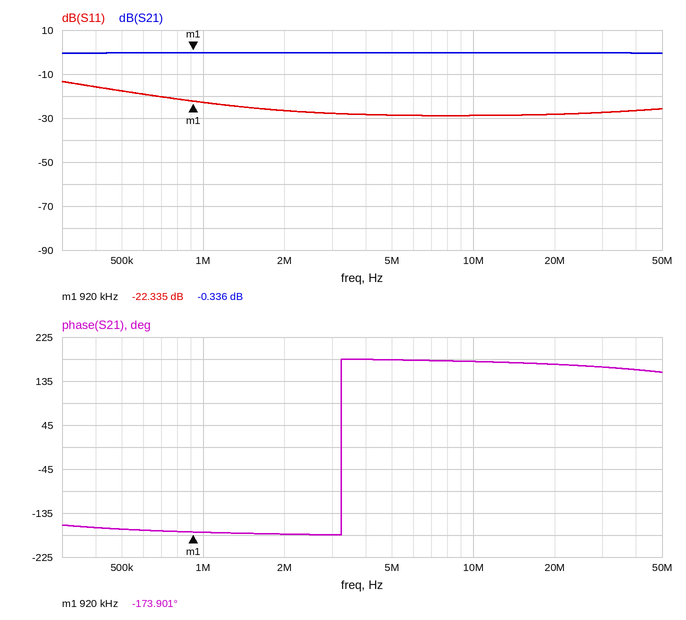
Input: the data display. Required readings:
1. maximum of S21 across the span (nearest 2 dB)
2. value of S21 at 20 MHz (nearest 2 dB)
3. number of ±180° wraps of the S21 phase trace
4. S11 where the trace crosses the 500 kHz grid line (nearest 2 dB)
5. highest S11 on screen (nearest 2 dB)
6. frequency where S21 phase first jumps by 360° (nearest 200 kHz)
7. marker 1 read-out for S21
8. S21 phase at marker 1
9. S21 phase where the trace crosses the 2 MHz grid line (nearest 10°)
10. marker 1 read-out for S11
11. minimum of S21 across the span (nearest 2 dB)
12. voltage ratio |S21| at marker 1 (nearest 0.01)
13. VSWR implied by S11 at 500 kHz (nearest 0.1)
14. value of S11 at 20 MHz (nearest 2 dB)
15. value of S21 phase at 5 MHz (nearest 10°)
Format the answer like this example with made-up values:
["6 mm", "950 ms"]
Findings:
["0 dB", "0 dB", "1", "-18 dB", "-14 dB", "3.2 MHz", "-0.336 dB", "-173.901°", "-180°", "-22.335 dB", "0 dB", "0.96", "1.3", "-28 dB", "180°"]
